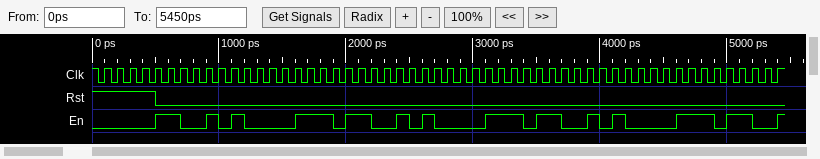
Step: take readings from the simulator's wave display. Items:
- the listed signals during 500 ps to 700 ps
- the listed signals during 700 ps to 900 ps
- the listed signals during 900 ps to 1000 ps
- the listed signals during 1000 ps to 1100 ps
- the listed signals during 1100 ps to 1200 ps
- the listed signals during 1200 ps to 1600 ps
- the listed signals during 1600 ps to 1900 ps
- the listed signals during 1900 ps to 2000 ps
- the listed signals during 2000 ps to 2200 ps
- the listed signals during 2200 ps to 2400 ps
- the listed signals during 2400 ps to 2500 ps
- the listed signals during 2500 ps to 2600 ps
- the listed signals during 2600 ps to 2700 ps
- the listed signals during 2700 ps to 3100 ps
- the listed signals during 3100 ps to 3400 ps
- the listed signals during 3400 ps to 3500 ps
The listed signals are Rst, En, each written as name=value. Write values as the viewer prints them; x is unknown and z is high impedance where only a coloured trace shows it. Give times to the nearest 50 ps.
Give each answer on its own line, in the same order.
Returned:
Rst=0, En=1
Rst=0, En=0
Rst=0, En=1
Rst=0, En=0
Rst=0, En=1
Rst=0, En=0
Rst=0, En=1
Rst=0, En=0
Rst=0, En=1
Rst=0, En=0
Rst=0, En=1
Rst=0, En=0
Rst=0, En=1
Rst=0, En=0
Rst=0, En=1
Rst=0, En=0
